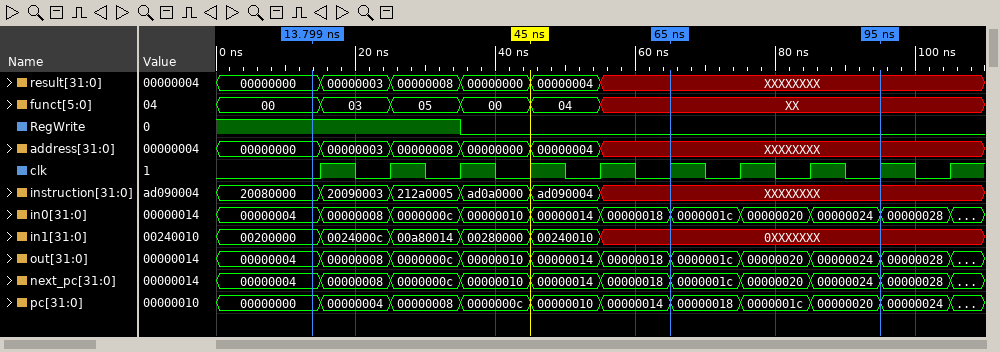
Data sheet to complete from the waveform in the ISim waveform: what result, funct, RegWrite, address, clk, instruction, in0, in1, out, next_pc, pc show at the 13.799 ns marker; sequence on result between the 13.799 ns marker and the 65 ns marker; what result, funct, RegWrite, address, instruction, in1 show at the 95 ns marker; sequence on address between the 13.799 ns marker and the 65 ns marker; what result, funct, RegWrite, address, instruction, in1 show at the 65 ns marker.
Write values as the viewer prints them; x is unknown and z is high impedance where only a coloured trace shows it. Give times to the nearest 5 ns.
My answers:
result=00000000, funct=00, RegWrite=1, address=00000000, clk=0, instruction=20080000, in0=00000004, in1=00200000, out=00000004, next_pc=00000004, pc=00000000
00000000, 00000003, 00000008, 00000000, 00000004, XXXXXXXX
result=XXXXXXXX, funct=XX, RegWrite=0, address=XXXXXXXX, instruction=XXXXXXXX, in1=0XXXXXXX
00000000, 00000003, 00000008, 00000000, 00000004, XXXXXXXX
result=XXXXXXXX, funct=XX, RegWrite=0, address=XXXXXXXX, instruction=XXXXXXXX, in1=0XXXXXXX
